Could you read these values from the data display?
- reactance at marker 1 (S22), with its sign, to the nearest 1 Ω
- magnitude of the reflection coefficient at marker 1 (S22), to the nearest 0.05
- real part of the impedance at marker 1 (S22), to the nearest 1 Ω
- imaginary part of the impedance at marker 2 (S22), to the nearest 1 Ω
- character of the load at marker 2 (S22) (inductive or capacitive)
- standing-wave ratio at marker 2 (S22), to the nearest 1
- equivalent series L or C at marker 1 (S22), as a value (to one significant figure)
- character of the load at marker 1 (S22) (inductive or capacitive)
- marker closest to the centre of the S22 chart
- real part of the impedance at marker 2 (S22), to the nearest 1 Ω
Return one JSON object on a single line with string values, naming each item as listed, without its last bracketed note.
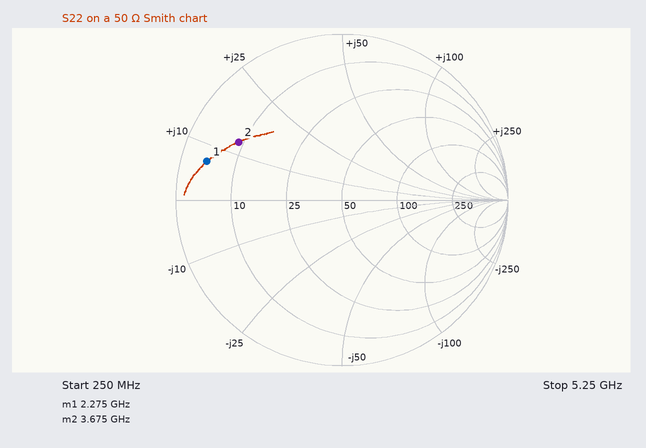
{"reactance at marker 1 (S22), with its sign, to the nearest 1 Ω": "+7 Ω", "magnitude of the reflection coefficient at marker 1 (S22), to the nearest 0.05": "0.85", "real part of the impedance at marker 1 (S22), to the nearest 1 Ω": "4 Ω", "imaginary part of the impedance at marker 2 (S22), to the nearest 1 Ω": "+13 Ω", "character of the load at marker 2 (S22)": "inductive", "standing-wave ratio at marker 2 (S22), to the nearest 1": "6", "equivalent series L or C at marker 1 (S22), as a value": "500 pH", "character of the load at marker 1 (S22)": "inductive", "marker closest to the centre of the S22 chart": "marker 2", "real part of the impedance at marker 2 (S22), to the nearest 1 Ω": "9 Ω"}
